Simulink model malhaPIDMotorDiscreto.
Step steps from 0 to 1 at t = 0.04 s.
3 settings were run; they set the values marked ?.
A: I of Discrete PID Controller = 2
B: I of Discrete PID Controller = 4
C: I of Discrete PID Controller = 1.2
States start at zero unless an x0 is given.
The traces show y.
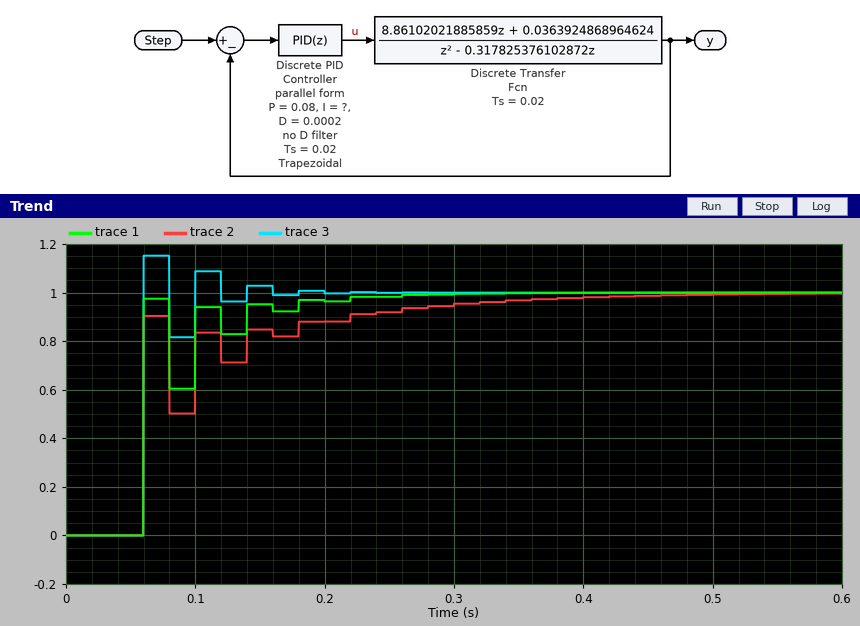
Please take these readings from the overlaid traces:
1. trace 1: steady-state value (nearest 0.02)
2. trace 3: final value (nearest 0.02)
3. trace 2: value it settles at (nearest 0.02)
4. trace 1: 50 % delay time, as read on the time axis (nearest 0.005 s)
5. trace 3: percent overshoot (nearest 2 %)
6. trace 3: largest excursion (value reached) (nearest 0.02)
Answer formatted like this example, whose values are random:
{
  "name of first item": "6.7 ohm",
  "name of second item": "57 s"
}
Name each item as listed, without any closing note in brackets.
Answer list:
{
  "trace 1: steady-state value": "1.00",
  "trace 3: final value": "1.00",
  "trace 2: value it settles at": "1.00",
  "trace 1: 50 % delay time, as read on the time axis": "0.060 s",
  "trace 3: percent overshoot": "16 %",
  "trace 3: largest excursion (value reached)": "1.16"
}
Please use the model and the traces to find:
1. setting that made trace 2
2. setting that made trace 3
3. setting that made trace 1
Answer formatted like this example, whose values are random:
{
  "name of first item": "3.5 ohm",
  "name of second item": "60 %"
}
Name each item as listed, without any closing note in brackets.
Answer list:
{
  "setting that made trace 2": "C",
  "setting that made trace 3": "B",
  "setting that made trace 1": "A"
}
